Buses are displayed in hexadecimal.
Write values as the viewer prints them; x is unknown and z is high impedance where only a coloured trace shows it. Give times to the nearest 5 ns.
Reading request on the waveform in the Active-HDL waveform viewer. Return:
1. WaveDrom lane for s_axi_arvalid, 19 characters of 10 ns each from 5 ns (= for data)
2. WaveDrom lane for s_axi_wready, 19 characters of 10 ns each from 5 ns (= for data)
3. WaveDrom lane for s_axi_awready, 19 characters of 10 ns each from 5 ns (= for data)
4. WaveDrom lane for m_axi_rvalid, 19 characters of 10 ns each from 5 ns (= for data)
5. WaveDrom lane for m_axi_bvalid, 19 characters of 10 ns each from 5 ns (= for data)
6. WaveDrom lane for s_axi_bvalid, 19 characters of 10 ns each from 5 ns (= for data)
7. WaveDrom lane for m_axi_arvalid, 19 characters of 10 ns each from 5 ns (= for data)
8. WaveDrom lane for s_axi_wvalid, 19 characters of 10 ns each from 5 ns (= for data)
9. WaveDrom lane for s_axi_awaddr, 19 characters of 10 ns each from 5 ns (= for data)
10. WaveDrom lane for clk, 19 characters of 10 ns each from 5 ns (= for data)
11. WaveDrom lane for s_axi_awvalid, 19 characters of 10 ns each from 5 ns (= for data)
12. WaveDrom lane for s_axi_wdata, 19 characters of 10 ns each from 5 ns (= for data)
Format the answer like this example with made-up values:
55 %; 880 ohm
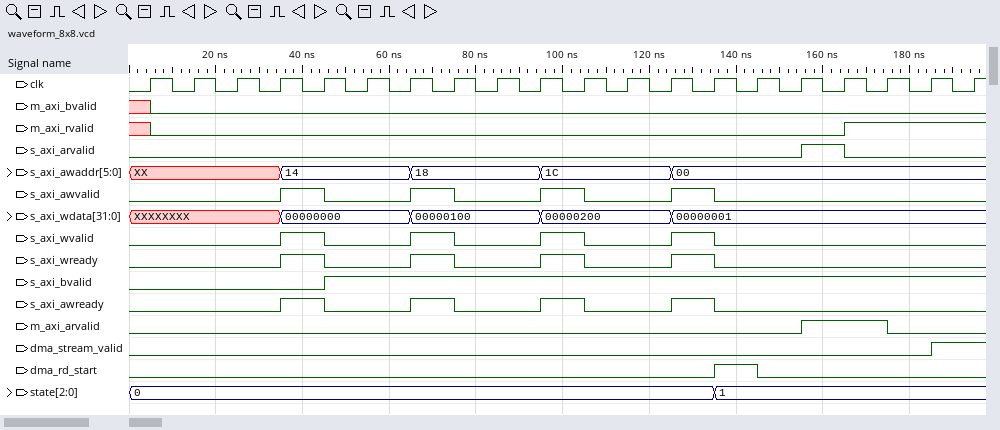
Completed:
{name: 's_axi_arvalid', wave: '0..............10..'}; {name: 's_axi_wready', wave: '0..10.10.10.10.....'}; {name: 's_axi_awready', wave: '0..10.10.10.10.....'}; {name: 'm_axi_rvalid', wave: '0...............1..'}; {name: 'm_axi_bvalid', wave: '0..................'}; {name: 's_axi_bvalid', wave: '0...1..............'}; {name: 'm_axi_arvalid', wave: '0..............1.0.'}; {name: 's_axi_wvalid', wave: '0..10.10.10.10.....'}; {name: 's_axi_awaddr', wave: 'x..=..=..=..=......', data: '14 18 1C 00'}; {name: 'clk', wave: 'p..................'}; {name: 's_axi_awvalid', wave: '0..10.10.10.10.....'}; {name: 's_axi_wdata', wave: 'x..=..=..=..=......', data: '00000000 00000100 00000200 00000001'}
